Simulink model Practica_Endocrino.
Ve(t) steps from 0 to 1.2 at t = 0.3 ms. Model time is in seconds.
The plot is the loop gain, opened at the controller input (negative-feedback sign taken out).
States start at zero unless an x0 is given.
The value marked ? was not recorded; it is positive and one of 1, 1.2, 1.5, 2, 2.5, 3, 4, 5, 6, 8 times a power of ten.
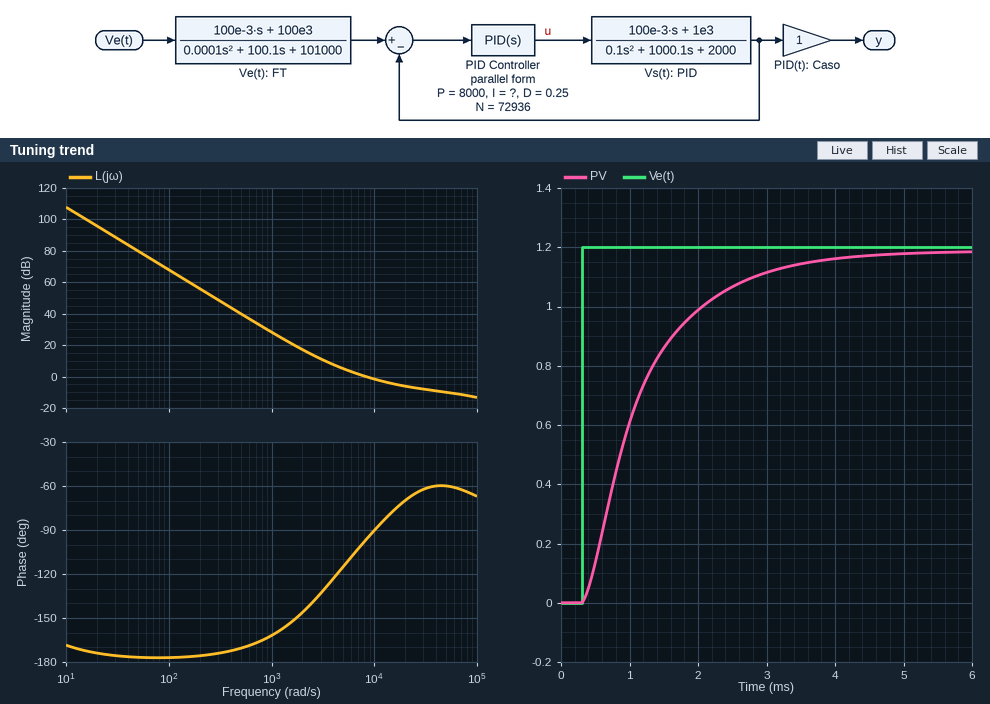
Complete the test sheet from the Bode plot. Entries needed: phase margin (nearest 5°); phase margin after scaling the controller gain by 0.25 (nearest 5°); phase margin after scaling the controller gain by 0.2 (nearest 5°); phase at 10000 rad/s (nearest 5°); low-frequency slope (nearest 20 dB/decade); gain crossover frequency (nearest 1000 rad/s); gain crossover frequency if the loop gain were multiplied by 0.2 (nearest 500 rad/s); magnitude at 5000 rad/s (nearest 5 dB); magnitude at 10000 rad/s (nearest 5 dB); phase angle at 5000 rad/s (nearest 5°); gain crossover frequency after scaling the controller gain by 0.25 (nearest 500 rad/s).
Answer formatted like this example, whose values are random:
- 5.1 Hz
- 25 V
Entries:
- 85°
- 45°
- 40°
- -90°
- -40 dB/decade
- 8000 rad/s
- 2500 rad/s
- 5 dB
- 0 dB
- -115°
- 3000 rad/s
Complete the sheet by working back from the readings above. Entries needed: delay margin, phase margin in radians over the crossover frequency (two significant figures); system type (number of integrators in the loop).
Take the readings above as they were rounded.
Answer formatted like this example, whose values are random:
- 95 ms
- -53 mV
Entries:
- 0.00019 s
- 2
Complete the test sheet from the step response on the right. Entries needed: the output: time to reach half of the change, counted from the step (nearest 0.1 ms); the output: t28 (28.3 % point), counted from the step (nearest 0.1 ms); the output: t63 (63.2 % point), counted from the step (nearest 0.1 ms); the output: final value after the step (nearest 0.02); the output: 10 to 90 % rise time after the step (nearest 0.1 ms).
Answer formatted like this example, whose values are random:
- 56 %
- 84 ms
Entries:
- 0.7 ms
- 0.4 ms
- 0.9 ms
- 1.18
- 2.0 ms
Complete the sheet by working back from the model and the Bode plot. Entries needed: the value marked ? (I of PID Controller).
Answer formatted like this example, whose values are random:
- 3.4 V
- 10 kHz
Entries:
- 2.5e+07
